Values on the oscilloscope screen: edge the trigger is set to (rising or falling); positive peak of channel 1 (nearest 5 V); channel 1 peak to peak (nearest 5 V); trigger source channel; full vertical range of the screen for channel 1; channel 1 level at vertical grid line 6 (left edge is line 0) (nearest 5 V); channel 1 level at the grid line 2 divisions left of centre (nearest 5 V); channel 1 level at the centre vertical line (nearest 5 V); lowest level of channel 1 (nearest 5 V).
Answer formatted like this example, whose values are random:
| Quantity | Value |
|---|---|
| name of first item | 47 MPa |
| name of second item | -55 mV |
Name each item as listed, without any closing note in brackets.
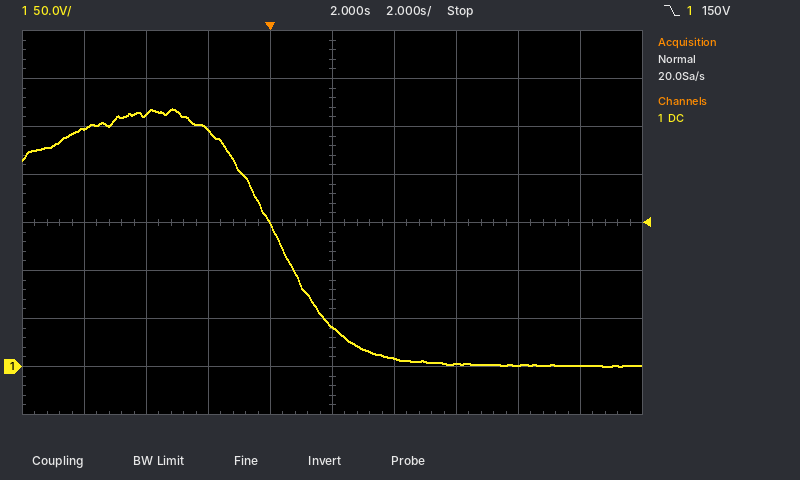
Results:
| Quantity | Value |
|---|---|
| edge the trigger is set to | falling |
| positive peak of channel 1 | 270 V |
| channel 1 peak to peak | 270 V |
| trigger source channel | channel 1 |
| full vertical range of the screen for channel 1 | 400 V |
| channel 1 level at vertical grid line 6 (left edge is line 0) | 10 V |
| channel 1 level at the grid line 2 divisions left of centre | 245 V |
| channel 1 level at the centre vertical line | 40 V |
| lowest level of channel 1 | 0 V |
